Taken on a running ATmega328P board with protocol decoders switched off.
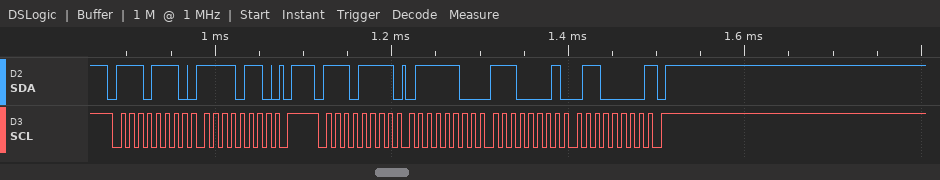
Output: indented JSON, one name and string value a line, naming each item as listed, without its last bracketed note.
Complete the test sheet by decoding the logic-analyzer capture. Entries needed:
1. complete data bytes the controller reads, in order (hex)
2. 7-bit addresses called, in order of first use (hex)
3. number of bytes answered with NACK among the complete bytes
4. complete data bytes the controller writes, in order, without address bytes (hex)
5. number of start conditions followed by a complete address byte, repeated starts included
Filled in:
{
  "complete data bytes the controller reads, in order": "7C E1 60",
  "7-bit addresses called, in order of first use": "0x77",
  "number of bytes answered with NACK among the complete bytes": "1",
  "complete data bytes the controller writes, in order, without address bytes": "F6",
  "number of start conditions followed by a complete address byte, repeated starts included": "2"
}
